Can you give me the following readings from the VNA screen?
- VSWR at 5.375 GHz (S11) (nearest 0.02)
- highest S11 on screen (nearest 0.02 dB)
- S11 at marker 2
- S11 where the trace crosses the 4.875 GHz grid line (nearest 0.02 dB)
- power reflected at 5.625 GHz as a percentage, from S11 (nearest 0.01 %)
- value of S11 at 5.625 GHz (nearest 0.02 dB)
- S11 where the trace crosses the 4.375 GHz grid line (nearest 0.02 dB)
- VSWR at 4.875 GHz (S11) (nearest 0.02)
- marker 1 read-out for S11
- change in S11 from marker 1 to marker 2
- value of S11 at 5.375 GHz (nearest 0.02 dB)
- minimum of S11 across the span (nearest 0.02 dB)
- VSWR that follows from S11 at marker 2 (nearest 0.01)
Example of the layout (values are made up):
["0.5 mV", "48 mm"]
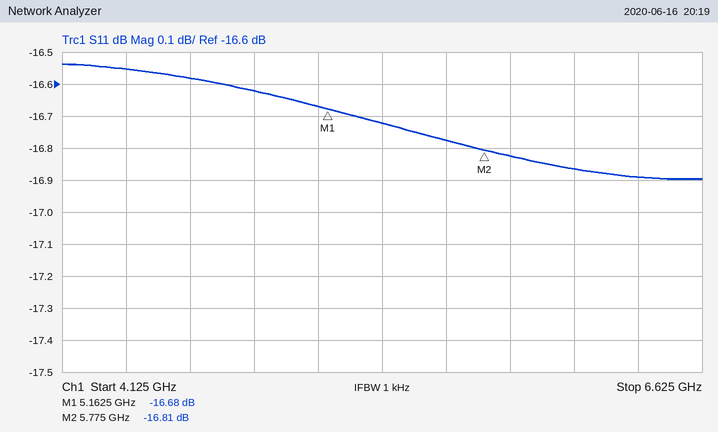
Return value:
["1.34", "-16.54 dB", "-16.81 dB", "-16.62 dB", "2.10 %", "-16.78 dB", "-16.56 dB", "1.34", "-16.68 dB", "-0.13 dB", "-16.72 dB", "-16.90 dB", "1.34"]
